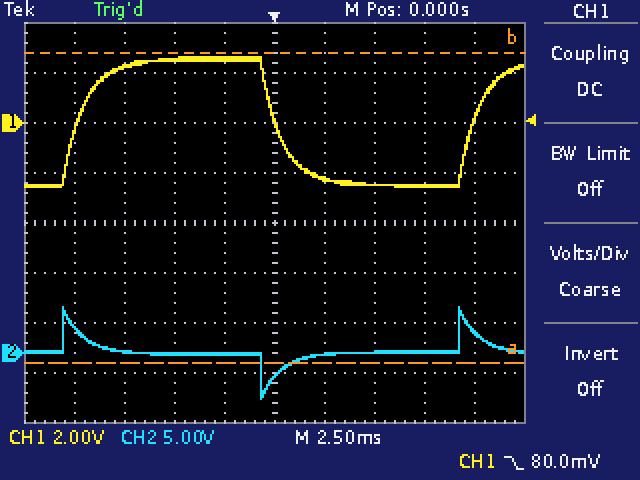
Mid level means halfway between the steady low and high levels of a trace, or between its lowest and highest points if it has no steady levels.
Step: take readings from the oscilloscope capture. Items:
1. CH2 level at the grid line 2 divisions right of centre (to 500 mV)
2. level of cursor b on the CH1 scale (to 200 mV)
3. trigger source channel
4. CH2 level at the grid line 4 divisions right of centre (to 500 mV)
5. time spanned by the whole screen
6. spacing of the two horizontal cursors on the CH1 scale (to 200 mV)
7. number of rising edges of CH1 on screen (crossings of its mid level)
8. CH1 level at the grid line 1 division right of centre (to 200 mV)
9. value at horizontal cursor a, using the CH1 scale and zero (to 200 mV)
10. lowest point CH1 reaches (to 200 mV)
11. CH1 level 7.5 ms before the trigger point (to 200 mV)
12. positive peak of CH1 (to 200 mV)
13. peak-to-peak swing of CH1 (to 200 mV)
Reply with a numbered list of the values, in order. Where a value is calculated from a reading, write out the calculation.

1. 0.0 V
2. 2.8 V
3. CH1
4. 2.0 V
5. 25 ms
6. 12.4 V
7. 2
8. -2.2 V
9. -9.6 V
10. -2.6 V
11. 2.2 V
12. 2.6 V
13. 2.6 V − (-2.6 V) = 5.2 V
